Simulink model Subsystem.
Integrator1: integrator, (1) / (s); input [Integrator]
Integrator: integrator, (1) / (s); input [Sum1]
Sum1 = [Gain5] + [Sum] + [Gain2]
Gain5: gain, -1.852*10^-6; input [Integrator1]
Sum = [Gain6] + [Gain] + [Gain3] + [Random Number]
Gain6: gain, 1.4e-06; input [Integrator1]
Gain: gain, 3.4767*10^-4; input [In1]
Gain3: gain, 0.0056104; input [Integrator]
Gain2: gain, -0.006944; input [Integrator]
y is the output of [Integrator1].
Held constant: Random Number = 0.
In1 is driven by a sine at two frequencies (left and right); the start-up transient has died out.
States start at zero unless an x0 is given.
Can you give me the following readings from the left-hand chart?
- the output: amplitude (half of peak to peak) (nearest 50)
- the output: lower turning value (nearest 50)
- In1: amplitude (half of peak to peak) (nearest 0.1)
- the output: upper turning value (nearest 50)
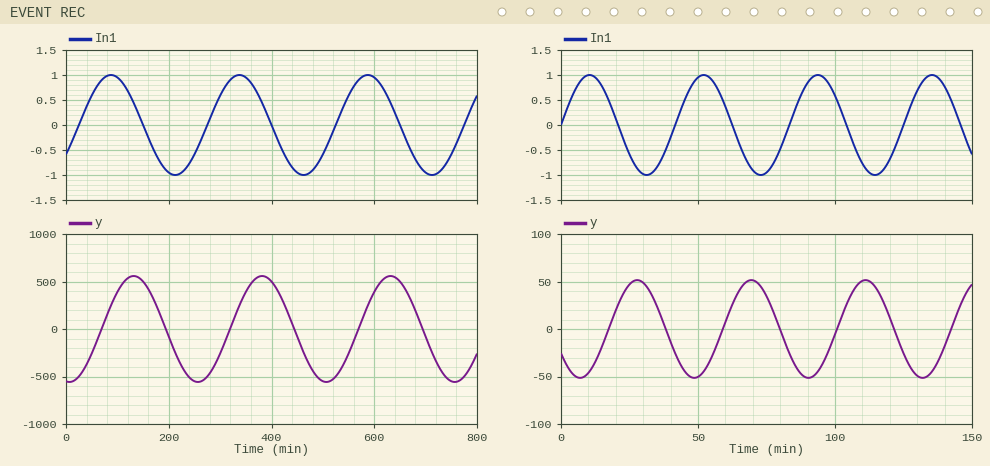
550
-550
1.0
550
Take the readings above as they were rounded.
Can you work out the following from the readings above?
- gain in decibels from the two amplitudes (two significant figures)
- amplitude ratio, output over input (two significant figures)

55 dB
550
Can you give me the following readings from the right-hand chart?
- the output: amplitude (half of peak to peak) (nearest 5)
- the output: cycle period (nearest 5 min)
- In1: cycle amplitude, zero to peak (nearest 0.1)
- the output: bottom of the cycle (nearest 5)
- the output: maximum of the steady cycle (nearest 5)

50
40 min
1.0
-50
50
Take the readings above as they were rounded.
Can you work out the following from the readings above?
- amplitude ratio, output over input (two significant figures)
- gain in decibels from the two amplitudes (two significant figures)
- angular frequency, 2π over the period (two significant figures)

50
34 dB
0.16 rad/min
